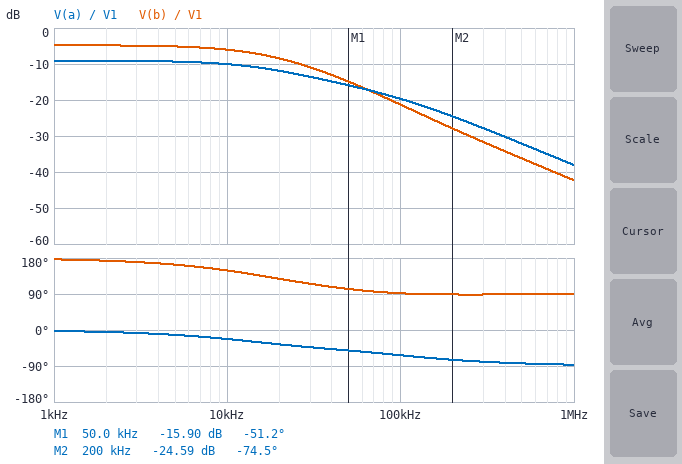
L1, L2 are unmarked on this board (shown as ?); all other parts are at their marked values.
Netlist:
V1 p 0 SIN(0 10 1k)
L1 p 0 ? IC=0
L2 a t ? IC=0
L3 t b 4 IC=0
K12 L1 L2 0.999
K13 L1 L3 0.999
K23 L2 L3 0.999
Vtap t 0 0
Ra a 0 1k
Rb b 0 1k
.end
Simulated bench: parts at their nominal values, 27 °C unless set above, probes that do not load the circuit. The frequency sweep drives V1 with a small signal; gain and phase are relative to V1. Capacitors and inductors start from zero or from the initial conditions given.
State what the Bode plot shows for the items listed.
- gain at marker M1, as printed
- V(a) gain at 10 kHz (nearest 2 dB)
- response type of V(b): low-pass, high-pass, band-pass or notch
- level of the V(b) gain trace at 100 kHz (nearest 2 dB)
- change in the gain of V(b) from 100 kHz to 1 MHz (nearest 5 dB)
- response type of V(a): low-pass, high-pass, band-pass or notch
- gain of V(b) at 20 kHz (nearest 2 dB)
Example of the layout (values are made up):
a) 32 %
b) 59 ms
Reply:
a) -15.90 dB
b) -10 dB
c) low-pass
d) -22 dB
e) -20 dB
f) low-pass
g) -8 dB
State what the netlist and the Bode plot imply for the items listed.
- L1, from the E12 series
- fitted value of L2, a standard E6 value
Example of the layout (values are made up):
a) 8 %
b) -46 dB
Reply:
a) 12 H
b) 1.5 H
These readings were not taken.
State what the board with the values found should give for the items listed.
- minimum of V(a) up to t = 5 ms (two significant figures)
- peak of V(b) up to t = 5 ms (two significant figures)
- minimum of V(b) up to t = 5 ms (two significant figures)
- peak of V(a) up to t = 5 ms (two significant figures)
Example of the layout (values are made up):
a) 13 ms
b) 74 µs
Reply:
a) -3.5 V
b) 5.8 V
c) -5.8 V
d) 3.5 V
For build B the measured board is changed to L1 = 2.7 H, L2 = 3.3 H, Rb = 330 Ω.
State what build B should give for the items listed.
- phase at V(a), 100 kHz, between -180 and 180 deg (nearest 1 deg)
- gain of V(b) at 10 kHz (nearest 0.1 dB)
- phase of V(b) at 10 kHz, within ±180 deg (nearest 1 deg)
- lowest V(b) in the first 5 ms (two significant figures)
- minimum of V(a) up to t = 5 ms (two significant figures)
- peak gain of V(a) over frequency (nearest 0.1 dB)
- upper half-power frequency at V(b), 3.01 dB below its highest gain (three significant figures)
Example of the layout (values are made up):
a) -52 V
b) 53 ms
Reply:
a) -75 deg
b) -4.2 dB
c) 117 deg
d) -12 V
e) -11 V
f) 0.9 dB
g) 5.98 kHz
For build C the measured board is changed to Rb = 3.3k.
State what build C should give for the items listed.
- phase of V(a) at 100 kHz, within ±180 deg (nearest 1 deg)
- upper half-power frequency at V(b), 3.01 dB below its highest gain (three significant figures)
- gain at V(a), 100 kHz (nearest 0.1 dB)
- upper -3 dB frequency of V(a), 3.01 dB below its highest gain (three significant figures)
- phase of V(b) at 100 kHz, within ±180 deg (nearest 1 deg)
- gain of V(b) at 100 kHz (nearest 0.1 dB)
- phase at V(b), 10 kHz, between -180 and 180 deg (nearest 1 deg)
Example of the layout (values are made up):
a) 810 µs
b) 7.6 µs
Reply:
a) -71 deg
b) 40.0 kHz
c) -18.2 dB
d) 38.3 kHz
e) 115 deg
f) -13.1 dB
g) 166 deg
